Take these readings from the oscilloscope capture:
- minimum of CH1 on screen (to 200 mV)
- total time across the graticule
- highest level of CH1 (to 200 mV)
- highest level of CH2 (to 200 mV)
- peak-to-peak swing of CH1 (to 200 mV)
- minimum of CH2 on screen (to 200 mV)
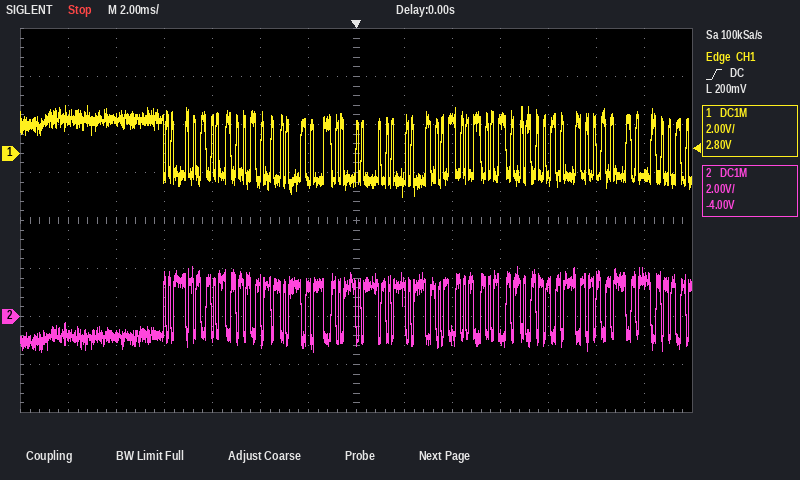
-1.8 V
28 ms
2.0 V
2.0 V
3.8 V
-1.4 V
